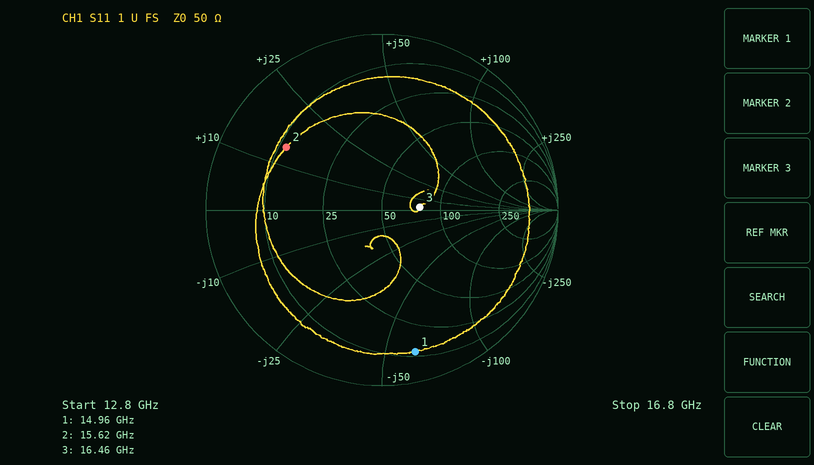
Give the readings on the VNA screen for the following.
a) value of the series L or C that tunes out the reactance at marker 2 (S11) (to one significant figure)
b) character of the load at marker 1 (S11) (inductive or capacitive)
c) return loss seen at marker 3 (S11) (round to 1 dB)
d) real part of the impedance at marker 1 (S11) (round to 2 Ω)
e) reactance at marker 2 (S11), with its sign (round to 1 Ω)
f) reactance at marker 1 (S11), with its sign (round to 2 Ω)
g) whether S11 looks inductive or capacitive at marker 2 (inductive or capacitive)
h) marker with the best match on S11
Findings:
700 fF
capacitive
13 dB
12 Ω
+14 Ω
-62 Ω
inductive
marker 3
